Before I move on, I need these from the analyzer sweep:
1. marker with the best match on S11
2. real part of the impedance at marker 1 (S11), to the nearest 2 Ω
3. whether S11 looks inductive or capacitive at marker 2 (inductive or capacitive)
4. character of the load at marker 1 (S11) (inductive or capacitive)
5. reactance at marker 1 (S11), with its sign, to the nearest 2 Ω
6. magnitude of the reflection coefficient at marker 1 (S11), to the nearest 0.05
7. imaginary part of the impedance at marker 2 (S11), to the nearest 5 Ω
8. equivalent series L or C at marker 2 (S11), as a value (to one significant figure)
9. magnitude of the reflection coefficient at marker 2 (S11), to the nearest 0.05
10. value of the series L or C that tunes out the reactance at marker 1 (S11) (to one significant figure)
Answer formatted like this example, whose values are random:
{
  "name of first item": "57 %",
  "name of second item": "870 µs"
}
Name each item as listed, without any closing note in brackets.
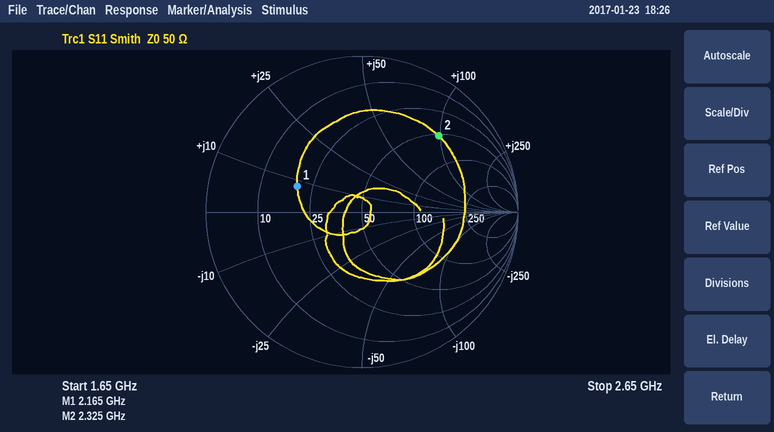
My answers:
{
  "marker with the best match on S11": "marker 1",
  "real part of the impedance at marker 1 (S11), to the nearest 2 Ω": "20 Ω",
  "whether S11 looks inductive or capacitive at marker 2": "inductive",
  "character of the load at marker 1 (S11)": "inductive",
  "reactance at marker 1 (S11), with its sign, to the nearest 2 Ω": "+8 Ω",
  "magnitude of the reflection coefficient at marker 1 (S11), to the nearest 0.05": "0.45",
  "imaginary part of the impedance at marker 2 (S11), to the nearest 5 Ω": "+100 Ω",
  "equivalent series L or C at marker 2 (S11), as a value": "7 nH",
  "magnitude of the reflection coefficient at marker 2 (S11), to the nearest 0.05": "0.70",
  "value of the series L or C that tunes out the reactance at marker 1 (S11)": "9 pF"
}
